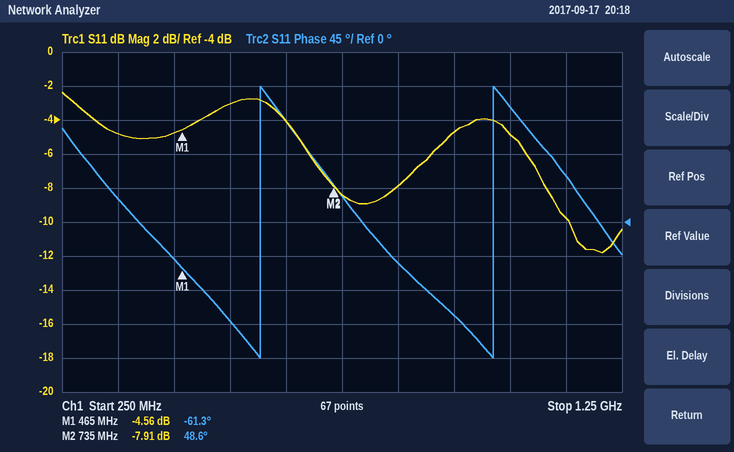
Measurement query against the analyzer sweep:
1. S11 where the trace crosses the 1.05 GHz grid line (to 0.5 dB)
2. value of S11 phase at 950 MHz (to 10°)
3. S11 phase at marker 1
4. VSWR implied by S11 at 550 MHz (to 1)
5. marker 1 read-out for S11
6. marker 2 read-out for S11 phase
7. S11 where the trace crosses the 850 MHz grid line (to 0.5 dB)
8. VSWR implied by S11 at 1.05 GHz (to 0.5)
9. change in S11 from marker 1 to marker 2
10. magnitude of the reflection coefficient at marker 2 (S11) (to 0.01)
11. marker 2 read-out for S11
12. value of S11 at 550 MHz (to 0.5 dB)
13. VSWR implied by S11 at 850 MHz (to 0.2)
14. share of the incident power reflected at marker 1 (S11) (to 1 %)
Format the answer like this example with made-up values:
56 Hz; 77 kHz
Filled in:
-5.0 dB; -120°; -61.3°; 6; -4.56 dB; 48.6°; -8.0 dB; 3.5; -3.35 dB; 0.40; -7.91 dB; -3.0 dB; 2.4; 35 %
